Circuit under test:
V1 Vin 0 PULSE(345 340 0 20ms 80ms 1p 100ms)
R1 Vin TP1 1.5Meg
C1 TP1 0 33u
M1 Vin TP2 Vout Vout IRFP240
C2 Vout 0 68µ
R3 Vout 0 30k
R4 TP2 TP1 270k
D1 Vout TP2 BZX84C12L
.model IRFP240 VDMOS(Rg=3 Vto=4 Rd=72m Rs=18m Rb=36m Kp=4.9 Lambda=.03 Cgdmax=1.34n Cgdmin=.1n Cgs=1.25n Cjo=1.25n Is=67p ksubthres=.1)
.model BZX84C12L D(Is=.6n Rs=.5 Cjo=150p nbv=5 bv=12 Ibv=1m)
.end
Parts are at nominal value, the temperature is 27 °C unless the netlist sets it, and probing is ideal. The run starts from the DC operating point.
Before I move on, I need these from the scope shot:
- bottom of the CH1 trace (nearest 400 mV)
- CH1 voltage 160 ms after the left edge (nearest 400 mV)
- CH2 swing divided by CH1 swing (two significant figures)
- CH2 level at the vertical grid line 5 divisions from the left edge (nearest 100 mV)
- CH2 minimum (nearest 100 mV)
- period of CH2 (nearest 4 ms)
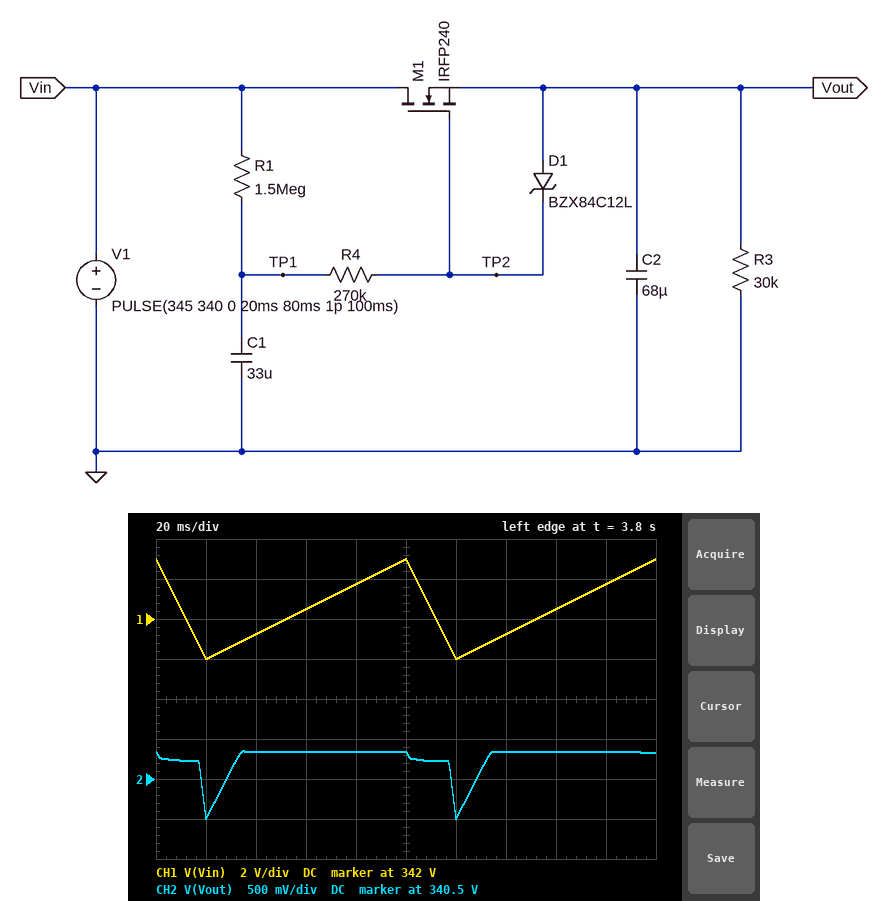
340.0 V
342.4 V
0.17
340.8 V
340.0 V
100 ms
